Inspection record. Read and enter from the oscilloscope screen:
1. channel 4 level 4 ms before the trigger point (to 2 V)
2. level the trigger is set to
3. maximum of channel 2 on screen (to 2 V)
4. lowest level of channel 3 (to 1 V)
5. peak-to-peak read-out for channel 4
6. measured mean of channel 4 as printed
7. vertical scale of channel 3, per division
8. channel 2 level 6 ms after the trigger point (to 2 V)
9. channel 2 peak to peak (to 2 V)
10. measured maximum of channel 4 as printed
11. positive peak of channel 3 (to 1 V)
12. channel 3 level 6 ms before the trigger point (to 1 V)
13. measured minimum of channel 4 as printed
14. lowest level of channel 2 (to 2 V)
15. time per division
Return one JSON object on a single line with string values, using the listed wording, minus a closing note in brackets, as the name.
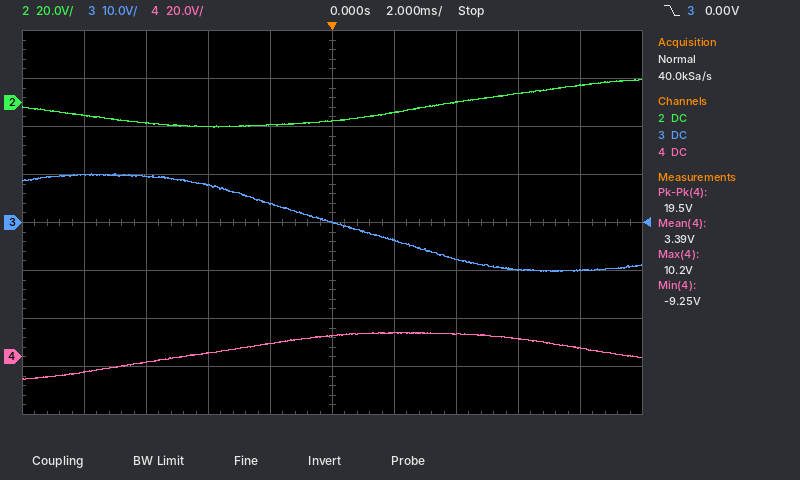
{"channel 4 level 4 ms before the trigger point": "2 V", "level the trigger is set to": "0.00 V", "maximum of channel 2 on screen": "10 V", "lowest level of channel 3": "-10 V", "peak-to-peak read-out for channel 4": "19.5 V", "measured mean of channel 4 as printed": "3.39 V", "vertical scale of channel 3, per division": "10 V", "channel 2 level 6 ms after the trigger point": "4 V", "channel 2 peak to peak": "20 V", "measured maximum of channel 4 as printed": "10.2 V", "positive peak of channel 3": "10 V", "channel 3 level 6 ms before the trigger point": "10 V", "measured minimum of channel 4 as printed": "-9.25 V", "lowest level of channel 2": "-10 V", "time per division": "2 ms"}
